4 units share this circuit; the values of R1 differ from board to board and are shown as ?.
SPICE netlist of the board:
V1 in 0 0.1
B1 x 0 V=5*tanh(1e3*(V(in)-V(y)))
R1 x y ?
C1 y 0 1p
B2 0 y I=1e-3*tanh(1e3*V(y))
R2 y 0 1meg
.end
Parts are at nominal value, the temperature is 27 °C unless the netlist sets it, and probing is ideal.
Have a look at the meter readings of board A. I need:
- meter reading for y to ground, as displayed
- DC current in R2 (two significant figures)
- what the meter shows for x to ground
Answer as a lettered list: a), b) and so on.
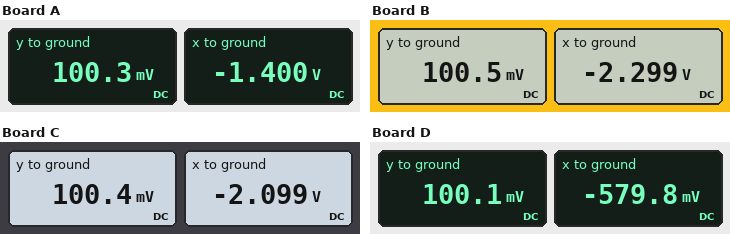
a) 100.3 mV
b) 100 nA
c) -1.400 V
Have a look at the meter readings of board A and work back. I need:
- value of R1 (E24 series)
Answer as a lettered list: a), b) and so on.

a) 1.5 kΩ
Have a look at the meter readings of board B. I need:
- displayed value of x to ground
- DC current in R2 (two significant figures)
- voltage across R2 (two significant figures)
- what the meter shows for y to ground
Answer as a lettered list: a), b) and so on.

a) -2.299 V
b) 100 nA
c) 100 mV
d) 100.5 mV
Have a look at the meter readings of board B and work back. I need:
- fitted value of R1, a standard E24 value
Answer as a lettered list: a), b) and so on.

a) 2.4 kΩ
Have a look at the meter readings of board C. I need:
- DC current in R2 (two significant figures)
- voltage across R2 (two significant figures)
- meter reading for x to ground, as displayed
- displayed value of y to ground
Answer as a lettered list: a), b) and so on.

a) 100 nA
b) 100 mV
c) -2.099 V
d) 100.4 mV
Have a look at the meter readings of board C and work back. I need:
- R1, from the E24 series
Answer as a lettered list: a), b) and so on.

a) 2.2 kΩ
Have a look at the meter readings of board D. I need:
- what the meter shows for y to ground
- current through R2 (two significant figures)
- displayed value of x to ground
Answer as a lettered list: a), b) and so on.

a) 100.1 mV
b) 100 nA
c) -579.8 mV
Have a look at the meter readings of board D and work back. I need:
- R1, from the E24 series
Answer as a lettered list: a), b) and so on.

a) 680 Ω
